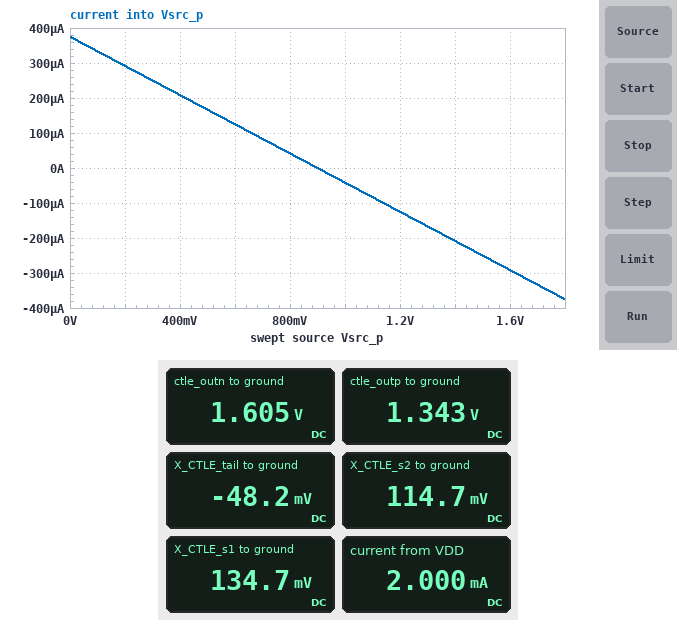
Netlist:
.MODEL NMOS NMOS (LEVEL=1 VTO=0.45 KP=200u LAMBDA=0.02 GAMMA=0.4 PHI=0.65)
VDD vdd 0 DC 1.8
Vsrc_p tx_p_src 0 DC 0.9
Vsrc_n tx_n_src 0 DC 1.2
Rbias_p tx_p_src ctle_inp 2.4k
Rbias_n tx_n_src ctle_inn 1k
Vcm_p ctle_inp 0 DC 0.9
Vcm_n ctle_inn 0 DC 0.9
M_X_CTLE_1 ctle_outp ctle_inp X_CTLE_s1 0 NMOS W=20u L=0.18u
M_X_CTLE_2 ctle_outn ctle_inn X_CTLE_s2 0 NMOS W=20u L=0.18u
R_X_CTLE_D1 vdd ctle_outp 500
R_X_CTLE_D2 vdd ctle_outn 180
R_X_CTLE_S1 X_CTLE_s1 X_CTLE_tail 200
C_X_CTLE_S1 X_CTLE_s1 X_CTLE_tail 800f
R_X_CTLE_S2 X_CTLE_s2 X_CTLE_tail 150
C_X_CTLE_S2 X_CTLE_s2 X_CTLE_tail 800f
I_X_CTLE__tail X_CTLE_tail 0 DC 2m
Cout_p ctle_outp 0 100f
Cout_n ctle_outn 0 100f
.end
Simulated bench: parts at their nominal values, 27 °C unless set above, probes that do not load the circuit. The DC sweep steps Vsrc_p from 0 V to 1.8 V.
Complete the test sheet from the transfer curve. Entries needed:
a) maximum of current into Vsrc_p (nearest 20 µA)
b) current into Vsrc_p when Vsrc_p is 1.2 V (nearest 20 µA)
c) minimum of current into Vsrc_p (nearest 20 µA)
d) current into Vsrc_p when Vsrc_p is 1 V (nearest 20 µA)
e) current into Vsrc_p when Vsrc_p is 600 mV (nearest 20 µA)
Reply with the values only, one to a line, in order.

380 µA
-120 µA
-380 µA
-40 µA
120 µA
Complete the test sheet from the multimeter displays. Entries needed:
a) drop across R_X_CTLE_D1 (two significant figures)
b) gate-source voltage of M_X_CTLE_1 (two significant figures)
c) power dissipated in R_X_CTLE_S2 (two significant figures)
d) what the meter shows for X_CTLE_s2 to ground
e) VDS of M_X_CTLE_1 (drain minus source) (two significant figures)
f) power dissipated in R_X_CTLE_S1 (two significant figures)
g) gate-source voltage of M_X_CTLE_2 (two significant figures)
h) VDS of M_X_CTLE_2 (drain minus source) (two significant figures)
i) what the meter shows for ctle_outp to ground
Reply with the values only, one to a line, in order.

460 mV
770 mV
180 µW
114.7 mV
1.2 V
170 µW
790 mV
1.5 V
1.343 V
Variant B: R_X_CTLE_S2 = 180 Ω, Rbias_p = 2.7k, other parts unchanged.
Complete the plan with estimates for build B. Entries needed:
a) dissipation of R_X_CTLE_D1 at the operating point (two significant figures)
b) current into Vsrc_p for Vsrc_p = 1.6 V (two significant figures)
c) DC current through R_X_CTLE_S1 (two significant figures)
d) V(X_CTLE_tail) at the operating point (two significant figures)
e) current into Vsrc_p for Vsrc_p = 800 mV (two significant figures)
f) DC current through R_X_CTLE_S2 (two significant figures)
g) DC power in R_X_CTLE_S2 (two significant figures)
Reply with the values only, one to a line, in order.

470 µW
-260 µA
970 µA
-65 mV
37 µA
1.0 mA
190 µW
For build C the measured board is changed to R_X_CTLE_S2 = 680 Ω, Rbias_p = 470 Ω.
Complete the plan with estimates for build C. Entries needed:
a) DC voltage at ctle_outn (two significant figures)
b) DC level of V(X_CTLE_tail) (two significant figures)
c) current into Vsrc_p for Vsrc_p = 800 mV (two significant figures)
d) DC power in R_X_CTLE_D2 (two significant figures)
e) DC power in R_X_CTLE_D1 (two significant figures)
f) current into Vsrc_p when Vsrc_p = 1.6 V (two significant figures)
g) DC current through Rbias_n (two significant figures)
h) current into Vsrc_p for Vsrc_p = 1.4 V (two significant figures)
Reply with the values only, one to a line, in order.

1.7 V
-210 mV
210 µA
60 µW
1.0 mW
-1.5 mA
300 µA
-1.1 mA
